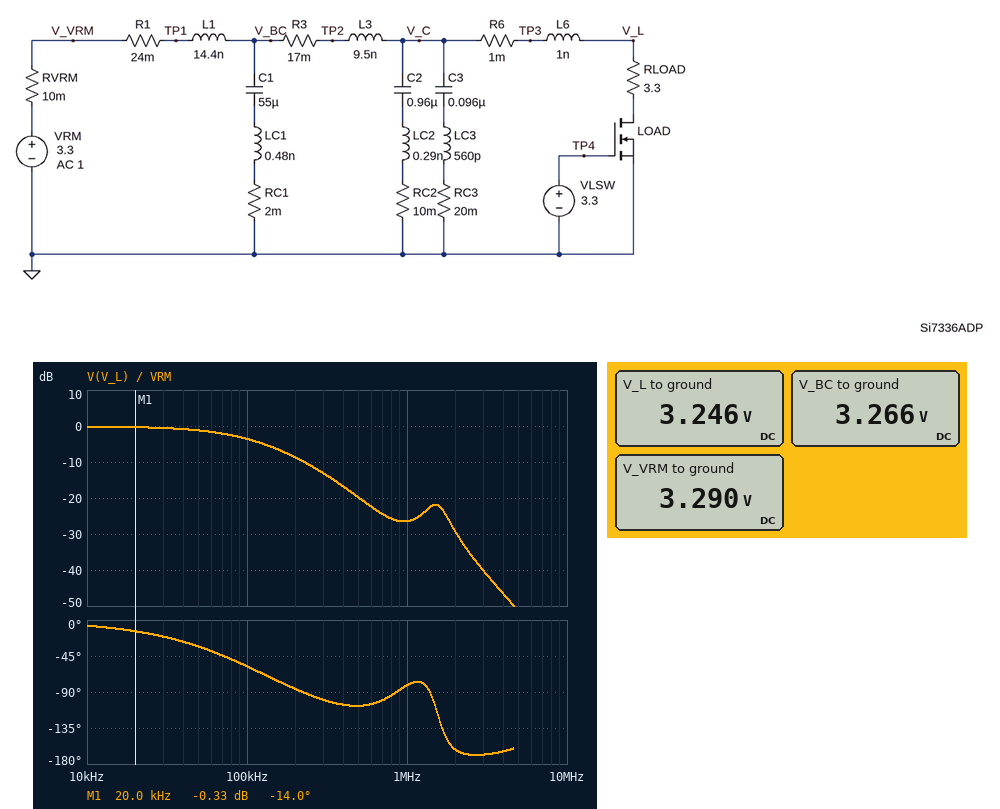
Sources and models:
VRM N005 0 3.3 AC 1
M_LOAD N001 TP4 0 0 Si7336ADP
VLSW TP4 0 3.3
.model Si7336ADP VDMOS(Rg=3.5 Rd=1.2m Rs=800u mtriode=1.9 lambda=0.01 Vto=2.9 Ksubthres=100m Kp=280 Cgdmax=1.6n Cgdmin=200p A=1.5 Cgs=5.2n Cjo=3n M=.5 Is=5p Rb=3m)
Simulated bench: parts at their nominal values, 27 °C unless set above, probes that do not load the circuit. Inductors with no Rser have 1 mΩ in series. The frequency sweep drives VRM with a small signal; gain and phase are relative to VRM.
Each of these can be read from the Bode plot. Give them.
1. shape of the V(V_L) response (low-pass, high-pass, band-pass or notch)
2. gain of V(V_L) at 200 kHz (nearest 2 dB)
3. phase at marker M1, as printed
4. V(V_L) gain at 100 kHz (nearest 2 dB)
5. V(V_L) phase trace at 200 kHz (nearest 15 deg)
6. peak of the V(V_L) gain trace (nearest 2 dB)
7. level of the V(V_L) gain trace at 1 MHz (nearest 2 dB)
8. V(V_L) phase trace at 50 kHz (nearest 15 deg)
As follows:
low-pass
-8 dB
-14.0 deg
-4 dB
-90 deg
0 dB
-26 dB
-30 deg
